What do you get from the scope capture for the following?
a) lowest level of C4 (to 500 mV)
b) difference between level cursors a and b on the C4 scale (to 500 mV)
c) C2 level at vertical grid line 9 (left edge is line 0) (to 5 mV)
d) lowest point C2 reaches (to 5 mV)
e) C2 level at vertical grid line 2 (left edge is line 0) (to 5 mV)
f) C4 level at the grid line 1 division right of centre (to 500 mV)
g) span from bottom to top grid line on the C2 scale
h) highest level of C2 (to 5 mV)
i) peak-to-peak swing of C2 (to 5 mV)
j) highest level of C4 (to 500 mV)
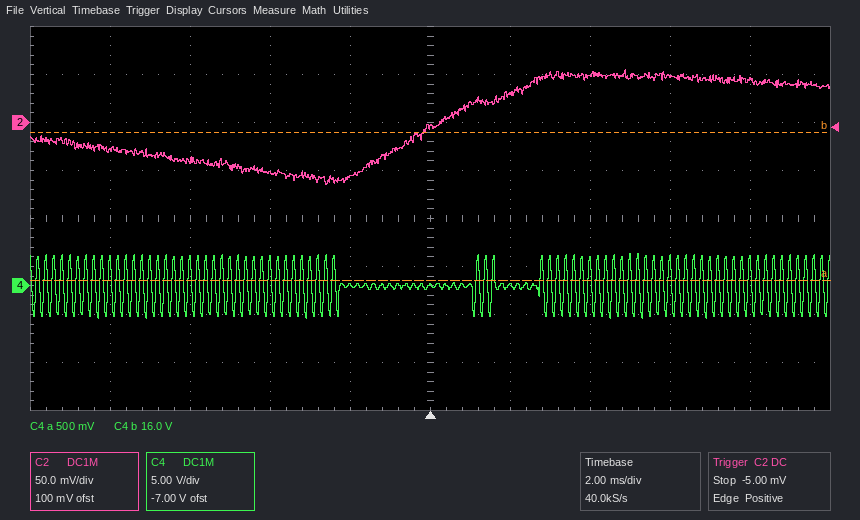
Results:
-3.5 V
15.5 V
45 mV
-65 mV
-40 mV
0.0 V
400 mV
55 mV
120 mV
3.5 V
